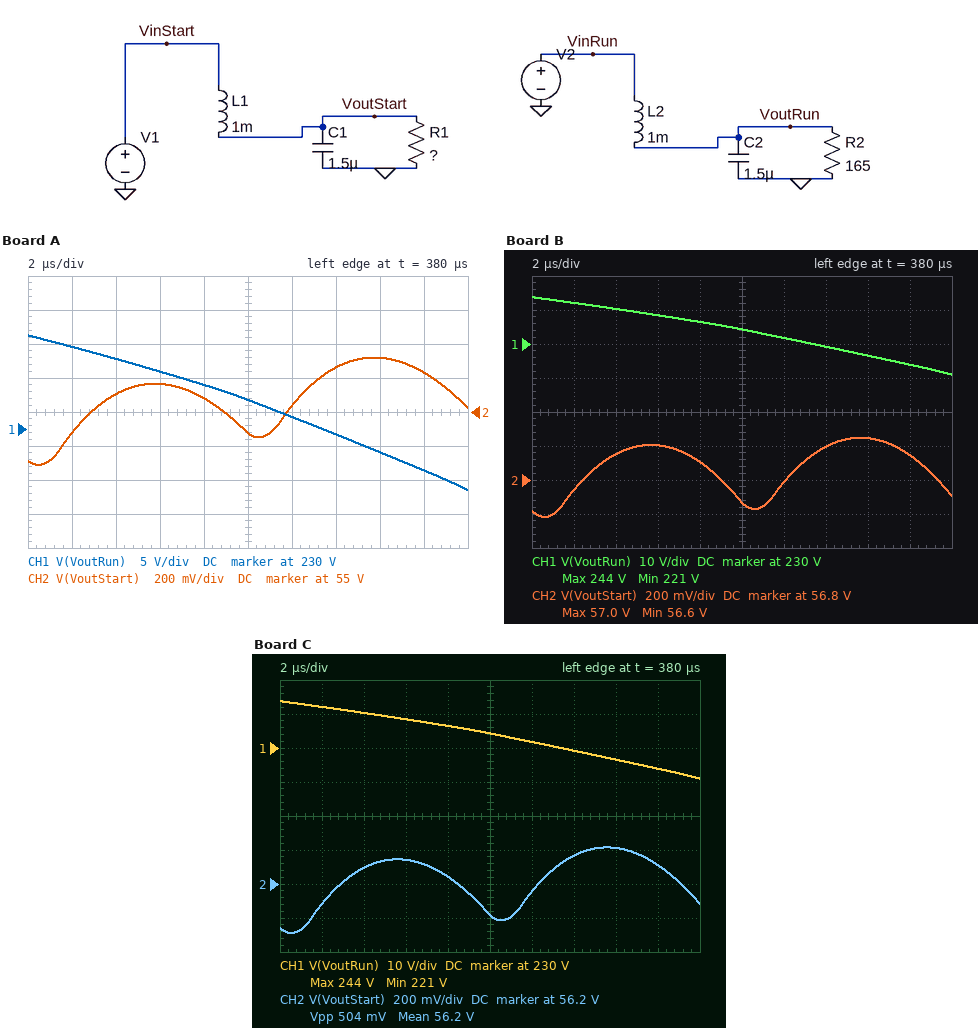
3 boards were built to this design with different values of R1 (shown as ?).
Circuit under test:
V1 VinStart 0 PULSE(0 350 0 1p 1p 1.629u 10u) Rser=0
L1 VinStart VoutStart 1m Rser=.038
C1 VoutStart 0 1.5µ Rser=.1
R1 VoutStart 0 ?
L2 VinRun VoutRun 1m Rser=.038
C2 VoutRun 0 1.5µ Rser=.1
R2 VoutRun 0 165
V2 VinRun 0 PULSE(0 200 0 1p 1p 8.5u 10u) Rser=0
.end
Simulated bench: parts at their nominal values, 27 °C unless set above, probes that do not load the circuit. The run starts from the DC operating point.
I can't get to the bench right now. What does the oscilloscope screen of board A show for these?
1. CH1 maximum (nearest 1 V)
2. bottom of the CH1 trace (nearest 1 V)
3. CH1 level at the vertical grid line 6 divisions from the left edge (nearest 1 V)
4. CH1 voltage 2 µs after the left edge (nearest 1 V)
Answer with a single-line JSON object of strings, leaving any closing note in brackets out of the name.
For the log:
{"CH1 maximum": "244 V", "bottom of the CH1 trace": "221 V", "CH1 level at the vertical grid line 6 divisions from the left edge": "232 V", "CH1 voltage 2 µs after the left edge": "242 V"}
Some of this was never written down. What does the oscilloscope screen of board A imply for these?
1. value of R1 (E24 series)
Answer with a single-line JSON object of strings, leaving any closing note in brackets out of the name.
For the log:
{"value of R1": "8.2 Ω"}
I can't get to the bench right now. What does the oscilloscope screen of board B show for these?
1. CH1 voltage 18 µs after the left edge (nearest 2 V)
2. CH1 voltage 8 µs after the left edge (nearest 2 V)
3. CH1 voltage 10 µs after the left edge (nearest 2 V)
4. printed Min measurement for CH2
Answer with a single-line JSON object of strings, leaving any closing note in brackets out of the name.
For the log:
{"CH1 voltage 18 µs after the left edge": "224 V", "CH1 voltage 8 µs after the left edge": "236 V", "CH1 voltage 10 µs after the left edge": "234 V", "printed Min measurement for CH2": "56.6 V"}
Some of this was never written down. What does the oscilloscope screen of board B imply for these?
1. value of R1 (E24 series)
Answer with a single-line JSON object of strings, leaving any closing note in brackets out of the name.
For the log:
{"value of R1": "22 Ω"}
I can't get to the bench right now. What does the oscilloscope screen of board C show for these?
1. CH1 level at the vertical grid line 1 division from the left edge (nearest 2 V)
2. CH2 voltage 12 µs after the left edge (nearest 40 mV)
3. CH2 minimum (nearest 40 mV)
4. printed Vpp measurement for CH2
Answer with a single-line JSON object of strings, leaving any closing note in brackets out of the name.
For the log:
{"CH1 level at the vertical grid line 1 division from the left edge": "242 V", "CH2 voltage 12 µs after the left edge": "56.16 V", "CH2 minimum": "55.92 V", "printed Vpp measurement for CH2": "504 mV"}
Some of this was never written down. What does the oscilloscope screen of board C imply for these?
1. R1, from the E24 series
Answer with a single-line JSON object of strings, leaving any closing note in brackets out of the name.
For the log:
{"R1, from the E24 series": "10 Ω"}
